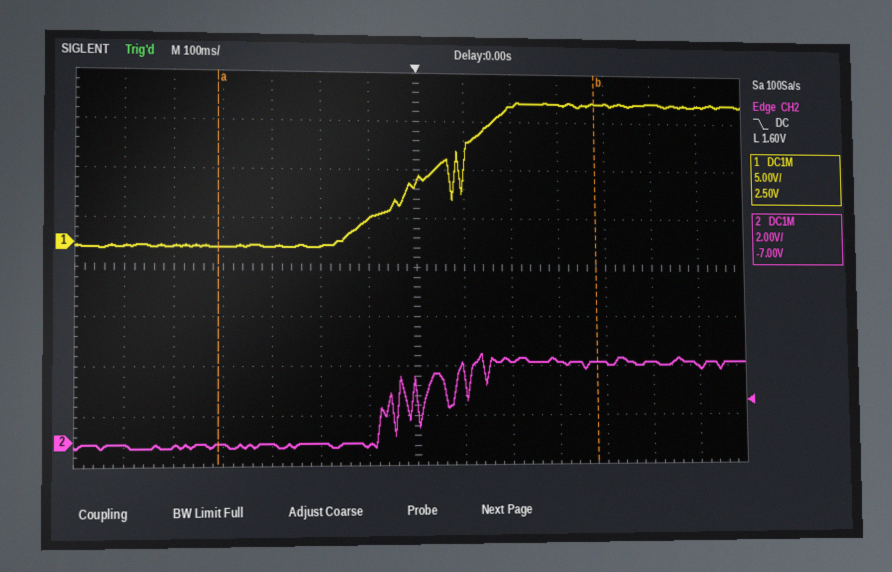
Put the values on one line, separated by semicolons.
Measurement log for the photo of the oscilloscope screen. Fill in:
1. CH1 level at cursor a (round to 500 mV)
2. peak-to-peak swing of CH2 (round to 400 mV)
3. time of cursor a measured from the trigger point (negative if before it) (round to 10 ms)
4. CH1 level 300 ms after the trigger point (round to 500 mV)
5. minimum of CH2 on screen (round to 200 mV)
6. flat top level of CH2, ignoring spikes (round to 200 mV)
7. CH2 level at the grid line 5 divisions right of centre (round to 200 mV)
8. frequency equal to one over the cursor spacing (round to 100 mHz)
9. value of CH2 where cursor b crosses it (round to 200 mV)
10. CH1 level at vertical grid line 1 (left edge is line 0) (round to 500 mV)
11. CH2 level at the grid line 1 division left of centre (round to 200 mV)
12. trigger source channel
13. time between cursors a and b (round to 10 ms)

-500 mV; 3.6 V; -410 ms; 14.5 V; -200 mV; 3.2 V; 3.2 V; 1.3 Hz; 3.2 V; -500 mV; -200 mV; CH2; 790 ms
